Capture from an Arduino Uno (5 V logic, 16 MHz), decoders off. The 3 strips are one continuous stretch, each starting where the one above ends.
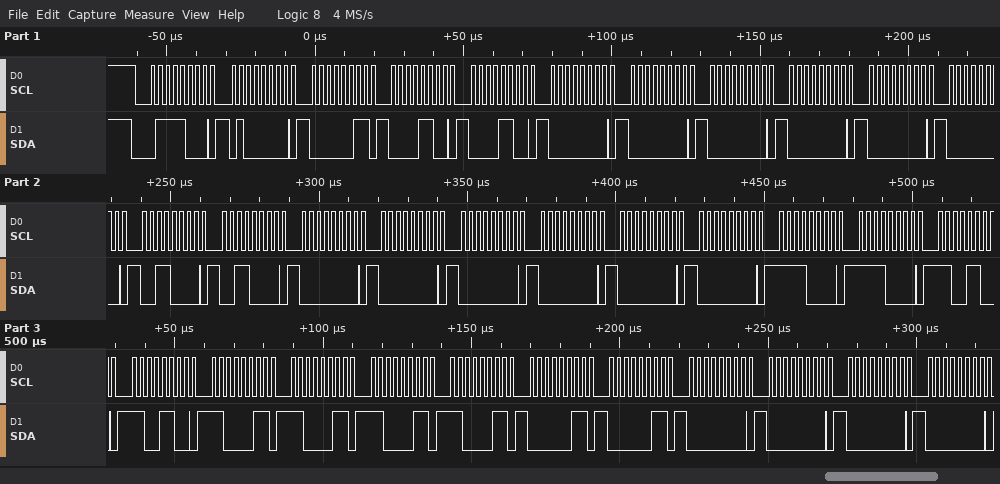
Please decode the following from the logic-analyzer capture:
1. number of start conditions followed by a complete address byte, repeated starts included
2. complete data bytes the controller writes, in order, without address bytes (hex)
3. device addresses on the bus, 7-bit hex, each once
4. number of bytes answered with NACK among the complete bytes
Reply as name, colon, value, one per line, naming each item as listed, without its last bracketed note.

number of start conditions followed by a complete address byte, repeated starts included: 1
complete data bytes the controller writes, in order, without address bytes: 40 03 0C 0C 00 00 00 00 00 00 30 30 00 00 00 00 00 00 F0 F0 CC CC C3 C3 C3 C3 03 03 00 00 00 00
device addresses on the bus, 7-bit hex, each once: 0x3C
number of bytes answered with NACK among the complete bytes: 0
